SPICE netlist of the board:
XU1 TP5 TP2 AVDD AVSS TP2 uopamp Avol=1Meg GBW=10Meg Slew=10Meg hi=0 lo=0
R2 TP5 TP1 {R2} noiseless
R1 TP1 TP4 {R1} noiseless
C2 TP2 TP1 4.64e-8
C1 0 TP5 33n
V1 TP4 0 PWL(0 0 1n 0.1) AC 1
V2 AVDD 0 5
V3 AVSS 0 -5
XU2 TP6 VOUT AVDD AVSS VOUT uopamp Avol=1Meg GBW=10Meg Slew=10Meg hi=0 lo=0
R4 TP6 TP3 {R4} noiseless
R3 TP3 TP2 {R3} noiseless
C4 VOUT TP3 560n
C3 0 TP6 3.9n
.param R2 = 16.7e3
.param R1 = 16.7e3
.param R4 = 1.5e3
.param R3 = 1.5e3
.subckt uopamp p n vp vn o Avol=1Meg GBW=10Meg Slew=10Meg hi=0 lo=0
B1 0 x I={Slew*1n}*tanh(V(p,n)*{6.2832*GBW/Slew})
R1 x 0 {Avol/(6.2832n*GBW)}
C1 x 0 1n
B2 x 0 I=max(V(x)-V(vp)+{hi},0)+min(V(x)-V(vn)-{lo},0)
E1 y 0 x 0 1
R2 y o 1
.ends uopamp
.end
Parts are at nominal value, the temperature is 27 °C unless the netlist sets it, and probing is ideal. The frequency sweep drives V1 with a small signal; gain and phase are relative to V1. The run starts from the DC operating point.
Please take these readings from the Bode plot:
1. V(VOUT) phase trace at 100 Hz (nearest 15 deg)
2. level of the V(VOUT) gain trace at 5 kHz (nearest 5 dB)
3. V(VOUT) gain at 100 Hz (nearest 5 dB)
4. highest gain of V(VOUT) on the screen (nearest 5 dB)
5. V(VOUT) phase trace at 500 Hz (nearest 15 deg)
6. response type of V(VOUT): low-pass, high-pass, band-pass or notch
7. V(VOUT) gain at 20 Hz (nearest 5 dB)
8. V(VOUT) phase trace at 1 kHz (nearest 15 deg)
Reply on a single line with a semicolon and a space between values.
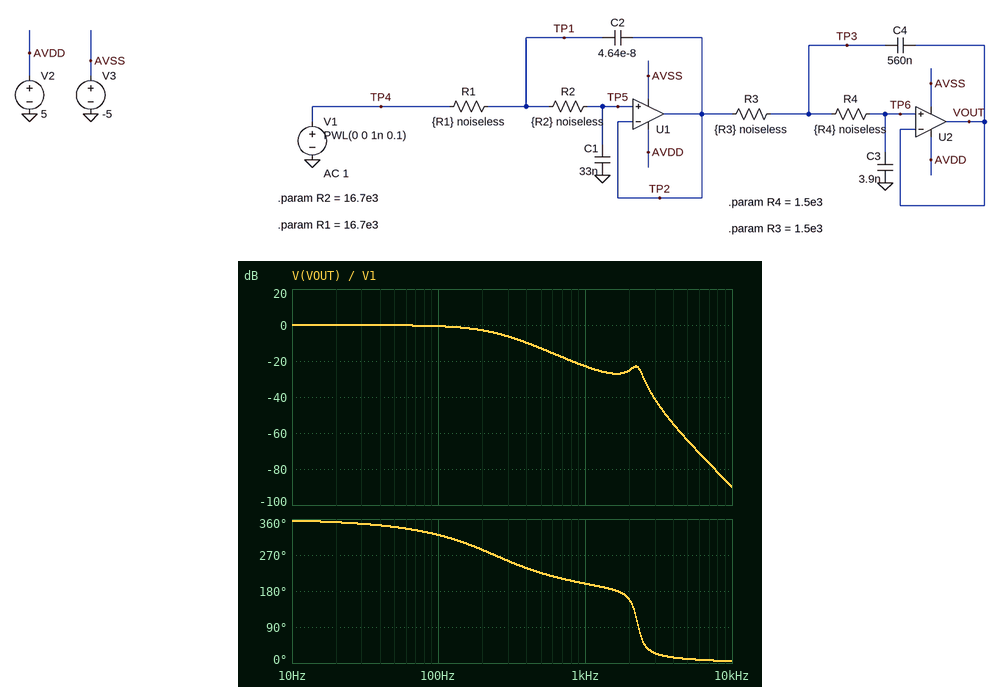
315 deg; -65 dB; 0 dB; 0 dB; 225 deg; low-pass; 0 dB; 195 deg
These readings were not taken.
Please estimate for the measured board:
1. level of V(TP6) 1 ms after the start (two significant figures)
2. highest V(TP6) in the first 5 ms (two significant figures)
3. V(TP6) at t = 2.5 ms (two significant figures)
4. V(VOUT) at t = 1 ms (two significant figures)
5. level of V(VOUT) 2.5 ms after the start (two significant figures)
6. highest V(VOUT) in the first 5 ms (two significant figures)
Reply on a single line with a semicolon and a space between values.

49 mV; 100 mV; 96 mV; 49 mV; 96 mV; 100 mV
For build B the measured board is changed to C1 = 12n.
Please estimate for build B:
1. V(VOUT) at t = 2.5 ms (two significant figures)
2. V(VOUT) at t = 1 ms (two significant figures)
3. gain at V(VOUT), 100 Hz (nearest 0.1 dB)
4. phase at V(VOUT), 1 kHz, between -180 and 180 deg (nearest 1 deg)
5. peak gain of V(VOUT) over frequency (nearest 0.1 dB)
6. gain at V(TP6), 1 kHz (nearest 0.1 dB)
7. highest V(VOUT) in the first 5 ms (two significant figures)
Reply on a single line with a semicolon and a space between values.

99 mV; 100 mV; 0.3 dB; -159 deg; 1.3 dB; -13.3 dB; 120 mV
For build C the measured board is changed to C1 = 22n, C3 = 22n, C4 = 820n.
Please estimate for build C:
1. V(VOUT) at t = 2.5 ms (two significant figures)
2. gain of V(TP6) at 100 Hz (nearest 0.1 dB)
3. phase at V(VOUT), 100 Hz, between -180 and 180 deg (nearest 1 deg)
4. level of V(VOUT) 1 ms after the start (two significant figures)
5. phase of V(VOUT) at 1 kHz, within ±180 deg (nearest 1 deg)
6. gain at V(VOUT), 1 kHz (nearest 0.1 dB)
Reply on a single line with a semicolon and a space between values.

110 mV; 0.1 dB; -30 deg; 69 mV; 59 deg; -18.3 dB
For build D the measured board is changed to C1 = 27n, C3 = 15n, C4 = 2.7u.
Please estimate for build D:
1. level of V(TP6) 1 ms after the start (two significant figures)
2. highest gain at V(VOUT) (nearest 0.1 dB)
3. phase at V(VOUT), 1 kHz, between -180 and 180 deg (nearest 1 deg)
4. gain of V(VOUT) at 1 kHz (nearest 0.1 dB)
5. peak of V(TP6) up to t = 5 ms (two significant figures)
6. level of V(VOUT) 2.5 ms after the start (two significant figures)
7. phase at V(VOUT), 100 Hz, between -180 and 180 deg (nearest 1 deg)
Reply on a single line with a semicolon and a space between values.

47 mV; 4.4 dB; 30 deg; -31.3 dB; 110 mV; 91 mV; -35 deg
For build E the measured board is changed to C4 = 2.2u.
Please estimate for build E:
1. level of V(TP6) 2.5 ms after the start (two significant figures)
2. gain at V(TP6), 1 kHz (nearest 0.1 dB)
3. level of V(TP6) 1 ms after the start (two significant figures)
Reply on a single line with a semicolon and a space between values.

98 mV; -12.6 dB; 51 mV
